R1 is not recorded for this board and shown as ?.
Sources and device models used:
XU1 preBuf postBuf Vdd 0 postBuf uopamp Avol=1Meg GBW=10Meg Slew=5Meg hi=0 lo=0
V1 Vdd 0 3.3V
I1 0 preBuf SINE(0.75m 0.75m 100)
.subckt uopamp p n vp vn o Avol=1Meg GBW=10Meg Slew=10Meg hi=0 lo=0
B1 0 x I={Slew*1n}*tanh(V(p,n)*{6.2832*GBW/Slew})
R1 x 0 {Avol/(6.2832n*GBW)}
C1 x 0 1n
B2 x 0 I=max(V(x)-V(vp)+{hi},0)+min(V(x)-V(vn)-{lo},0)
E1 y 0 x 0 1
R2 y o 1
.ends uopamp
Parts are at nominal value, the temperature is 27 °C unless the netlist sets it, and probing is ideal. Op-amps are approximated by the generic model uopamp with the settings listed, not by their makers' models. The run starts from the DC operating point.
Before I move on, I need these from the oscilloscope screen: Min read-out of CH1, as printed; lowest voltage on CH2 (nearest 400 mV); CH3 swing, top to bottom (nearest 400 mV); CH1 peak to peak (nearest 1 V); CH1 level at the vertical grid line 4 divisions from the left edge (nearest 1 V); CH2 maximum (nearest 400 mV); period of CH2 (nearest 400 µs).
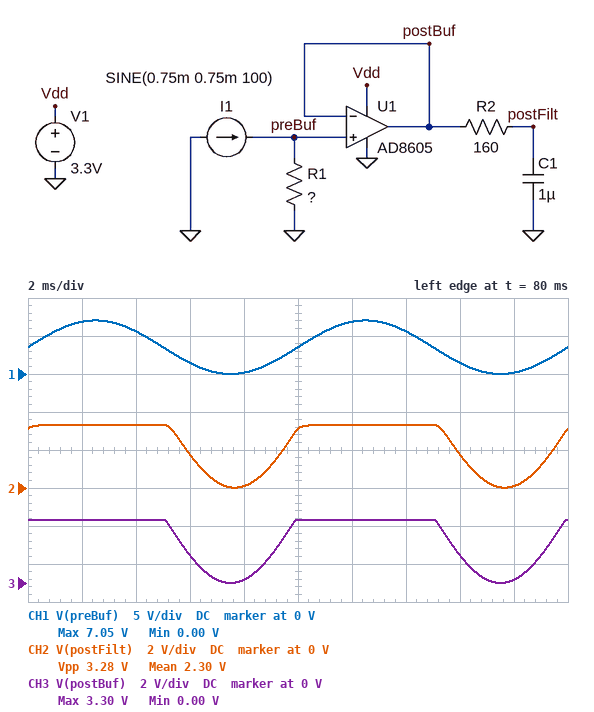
0.00 V
0 V
3.2 V
7 V
0 V
3.2 V
10.0 ms
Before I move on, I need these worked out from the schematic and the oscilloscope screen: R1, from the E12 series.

4.7 kΩ
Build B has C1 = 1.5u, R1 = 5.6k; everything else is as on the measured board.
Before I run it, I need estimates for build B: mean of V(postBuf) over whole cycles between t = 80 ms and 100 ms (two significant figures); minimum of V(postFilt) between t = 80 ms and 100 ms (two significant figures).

2.4 V
47 mV
